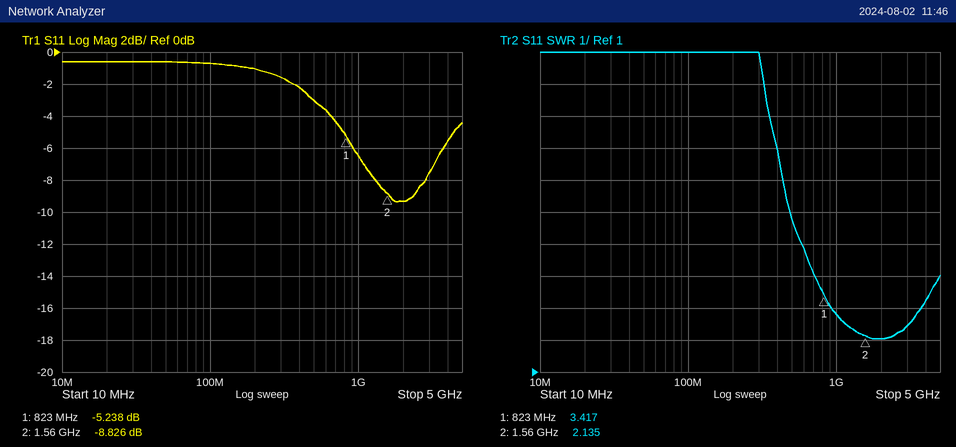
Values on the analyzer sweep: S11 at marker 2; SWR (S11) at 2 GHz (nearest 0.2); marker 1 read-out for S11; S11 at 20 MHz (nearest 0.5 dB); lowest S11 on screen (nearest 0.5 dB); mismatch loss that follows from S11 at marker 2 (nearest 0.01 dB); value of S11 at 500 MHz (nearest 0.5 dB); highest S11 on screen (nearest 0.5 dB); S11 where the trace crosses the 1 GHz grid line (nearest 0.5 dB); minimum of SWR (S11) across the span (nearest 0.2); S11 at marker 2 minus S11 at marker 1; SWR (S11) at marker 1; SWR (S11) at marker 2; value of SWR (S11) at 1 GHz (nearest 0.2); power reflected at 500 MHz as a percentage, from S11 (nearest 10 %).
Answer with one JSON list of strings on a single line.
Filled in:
["-8.826 dB", "2.0", "-5.238 dB", "-0.5 dB", "-9.5 dB", "0.61 dB", "-3.0 dB", "-0.5 dB", "-6.5 dB", "2.0", "-3.588 dB", "3.417", "2.135", "2.8", "50 %"]
